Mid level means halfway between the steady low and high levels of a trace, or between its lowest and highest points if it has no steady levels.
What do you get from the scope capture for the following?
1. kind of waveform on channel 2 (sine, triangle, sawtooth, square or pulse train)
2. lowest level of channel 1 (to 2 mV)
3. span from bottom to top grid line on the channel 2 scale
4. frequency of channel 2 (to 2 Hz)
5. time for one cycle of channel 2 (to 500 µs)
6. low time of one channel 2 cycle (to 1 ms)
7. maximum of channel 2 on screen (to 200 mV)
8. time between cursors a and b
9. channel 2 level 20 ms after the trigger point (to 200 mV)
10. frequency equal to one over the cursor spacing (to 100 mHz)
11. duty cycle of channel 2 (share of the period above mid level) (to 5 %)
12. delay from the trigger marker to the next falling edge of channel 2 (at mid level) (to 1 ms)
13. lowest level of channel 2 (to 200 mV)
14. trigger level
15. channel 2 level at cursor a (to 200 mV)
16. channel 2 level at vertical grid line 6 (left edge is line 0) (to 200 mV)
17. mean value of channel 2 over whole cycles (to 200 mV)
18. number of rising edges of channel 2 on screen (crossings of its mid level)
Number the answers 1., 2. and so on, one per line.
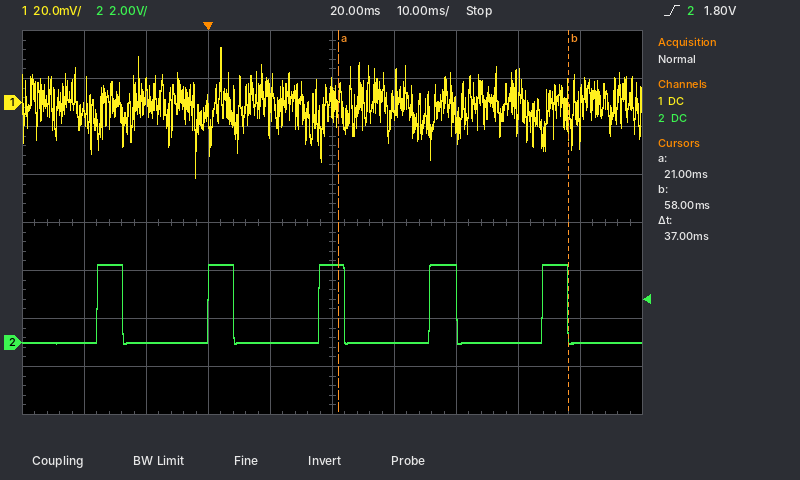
1. pulse train
2. -32 mV
3. 16 V
4. 56 Hz
5. 18.0 ms
6. 14 ms
7. 3.2 V
8. 37 ms
9. 3.2 V
10. 27.0 Hz
11. 25 %
12. 4 ms
13. 0.0 V
14. 1.80 V
15. 3.2 V
16. 0.0 V
17. 800 mV
18. 5
